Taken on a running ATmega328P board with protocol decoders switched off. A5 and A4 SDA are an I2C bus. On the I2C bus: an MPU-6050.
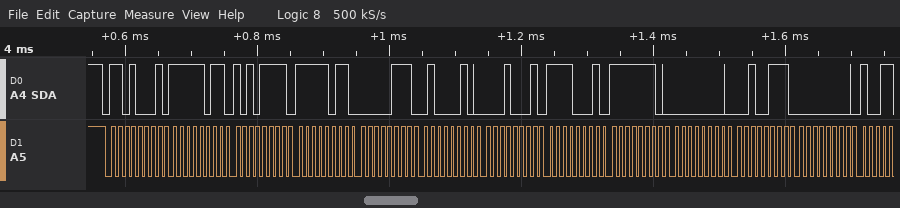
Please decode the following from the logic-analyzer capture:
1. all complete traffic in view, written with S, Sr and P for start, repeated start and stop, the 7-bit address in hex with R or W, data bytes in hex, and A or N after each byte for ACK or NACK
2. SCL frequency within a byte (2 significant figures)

S 68R A FB A AF A FB A 07 A 42 A 11 A F1 A FE A 00 A 27 A 00 A
100 kHz
